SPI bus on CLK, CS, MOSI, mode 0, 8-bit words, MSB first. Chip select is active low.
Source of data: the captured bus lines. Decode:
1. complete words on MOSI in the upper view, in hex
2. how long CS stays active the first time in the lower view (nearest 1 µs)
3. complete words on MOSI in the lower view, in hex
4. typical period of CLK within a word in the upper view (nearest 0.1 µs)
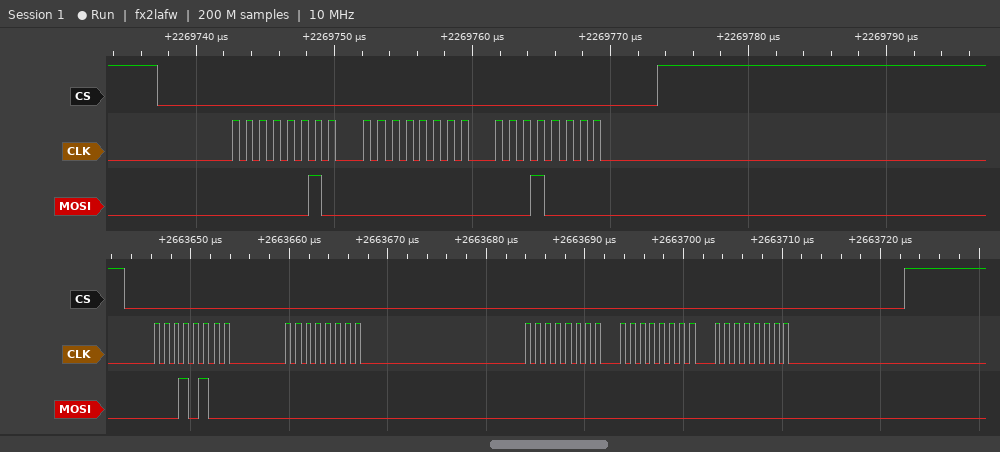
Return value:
02, 00, 10
79 µs
14, 00, 00, 00, 00
1 µs
